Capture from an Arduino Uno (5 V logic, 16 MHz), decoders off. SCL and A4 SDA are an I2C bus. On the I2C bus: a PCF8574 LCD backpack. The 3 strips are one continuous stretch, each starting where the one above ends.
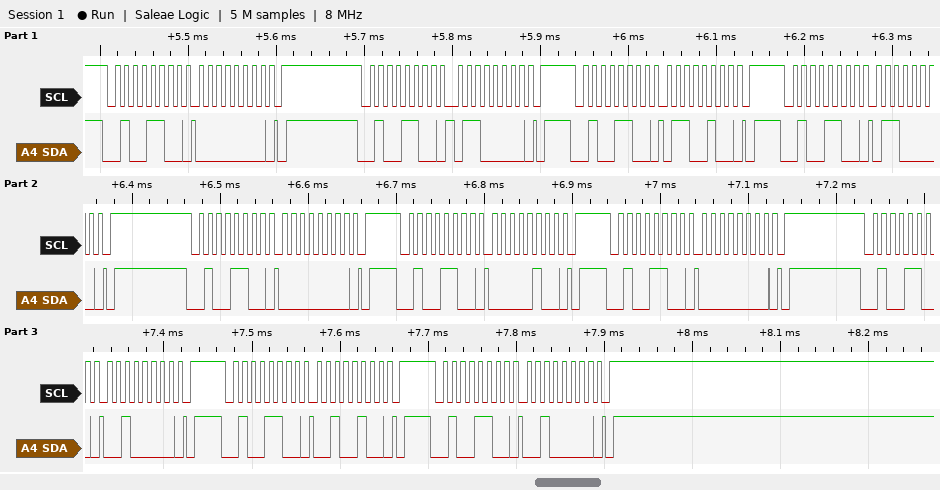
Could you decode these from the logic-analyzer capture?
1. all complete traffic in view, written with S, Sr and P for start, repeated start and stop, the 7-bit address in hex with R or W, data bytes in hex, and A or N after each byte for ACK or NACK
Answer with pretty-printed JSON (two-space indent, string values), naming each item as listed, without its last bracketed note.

{
  "all complete traffic in view, written with S, Sr and P for start, repeated start and stop, the 7-bit address in hex with R or W, data bytes in hex, and A or N after each byte for ACK or NACK": "S 26W A 00 A P S 26W A 60 A P S 26W A 64 A P S 26W A 60 A P S 26W A 00 A P S 26W A 04 A P S 26W A 00 A P S 26W A 20 A P S 26W A 24 A P S 26W A 20 A P"
}
